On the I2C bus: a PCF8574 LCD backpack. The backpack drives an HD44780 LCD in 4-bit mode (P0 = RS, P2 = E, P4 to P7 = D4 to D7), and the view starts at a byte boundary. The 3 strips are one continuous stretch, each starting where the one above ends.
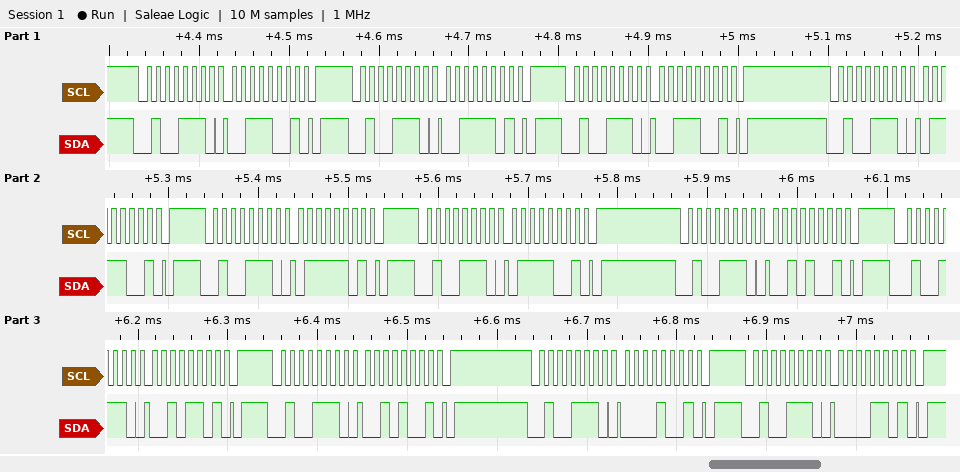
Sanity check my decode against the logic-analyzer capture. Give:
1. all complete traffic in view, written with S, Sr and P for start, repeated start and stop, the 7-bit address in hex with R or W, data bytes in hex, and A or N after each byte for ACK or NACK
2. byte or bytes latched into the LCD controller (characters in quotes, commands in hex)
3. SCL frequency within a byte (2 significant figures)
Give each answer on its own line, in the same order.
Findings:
S 27W A 39 A P S 27W A 3D A P S 27W A 39 A P S 27W A 79 A P S 27W A 7D A P S 27W A 79 A P S 27W A 29 A P S 27W A 2D A P S 27W A 29 A P S 27W A 09 A P S 27W A 0D A P
'7'
100 kHz
